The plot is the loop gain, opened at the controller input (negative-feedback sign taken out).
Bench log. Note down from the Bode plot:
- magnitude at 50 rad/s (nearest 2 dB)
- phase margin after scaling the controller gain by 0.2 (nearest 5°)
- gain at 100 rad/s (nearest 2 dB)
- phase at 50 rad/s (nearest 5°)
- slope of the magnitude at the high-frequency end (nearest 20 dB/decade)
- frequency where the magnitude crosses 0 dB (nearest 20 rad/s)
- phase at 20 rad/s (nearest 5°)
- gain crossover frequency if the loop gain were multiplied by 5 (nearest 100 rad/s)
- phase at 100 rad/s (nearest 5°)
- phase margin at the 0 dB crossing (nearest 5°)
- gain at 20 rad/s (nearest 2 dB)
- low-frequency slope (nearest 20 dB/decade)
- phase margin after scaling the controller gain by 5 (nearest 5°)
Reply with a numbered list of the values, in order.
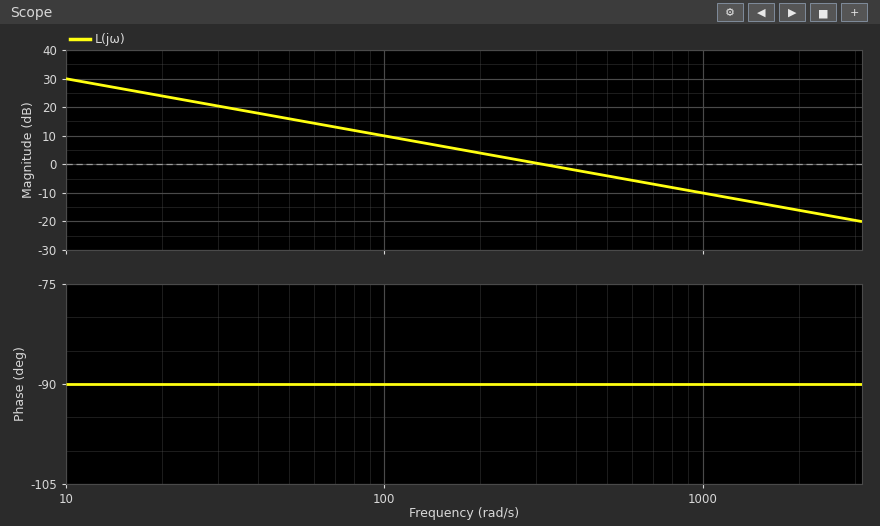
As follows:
1. 16 dB
2. 90°
3. 10 dB
4. -90°
5. -20 dB/decade
6. 320 rad/s
7. -90°
8. 1600 rad/s
9. -90°
10. 90°
11. 24 dB
12. -20 dB/decade
13. 90°
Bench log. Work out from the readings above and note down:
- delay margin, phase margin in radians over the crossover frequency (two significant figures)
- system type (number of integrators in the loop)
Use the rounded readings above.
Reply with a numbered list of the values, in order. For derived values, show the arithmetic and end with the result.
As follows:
1. 90 × π / 180 / 320 = 0.0049 s
2. 1
